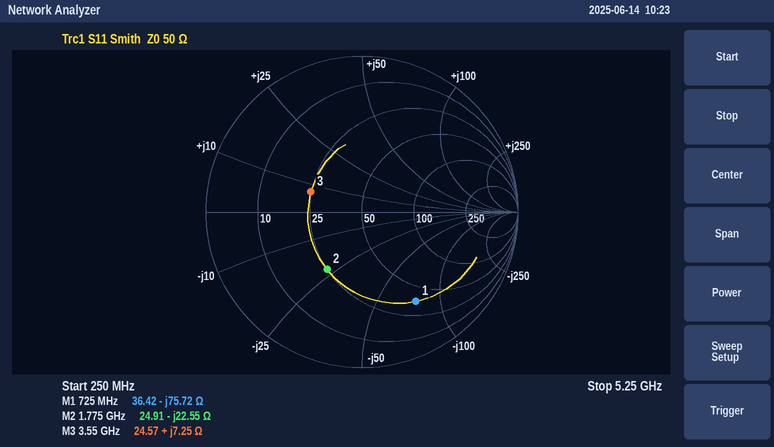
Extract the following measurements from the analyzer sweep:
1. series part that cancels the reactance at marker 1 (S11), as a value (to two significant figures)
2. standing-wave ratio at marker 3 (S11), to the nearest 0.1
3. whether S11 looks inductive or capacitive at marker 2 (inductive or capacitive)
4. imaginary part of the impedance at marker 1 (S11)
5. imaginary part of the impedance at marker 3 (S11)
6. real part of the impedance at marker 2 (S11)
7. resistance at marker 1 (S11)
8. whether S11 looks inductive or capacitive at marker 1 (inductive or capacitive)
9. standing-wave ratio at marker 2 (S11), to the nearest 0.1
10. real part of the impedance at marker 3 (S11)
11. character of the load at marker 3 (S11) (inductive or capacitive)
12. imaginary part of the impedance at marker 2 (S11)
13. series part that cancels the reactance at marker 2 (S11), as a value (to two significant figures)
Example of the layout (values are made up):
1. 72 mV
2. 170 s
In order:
1. 17 nH
2. 2.1
3. capacitive
4. -75.72 Ω
5. +7.25 Ω
6. 24.91 Ω
7. 36.42 Ω
8. capacitive
9. 2.5
10. 24.57 Ω
11. inductive
12. -22.55 Ω
13. 2.0 nH
